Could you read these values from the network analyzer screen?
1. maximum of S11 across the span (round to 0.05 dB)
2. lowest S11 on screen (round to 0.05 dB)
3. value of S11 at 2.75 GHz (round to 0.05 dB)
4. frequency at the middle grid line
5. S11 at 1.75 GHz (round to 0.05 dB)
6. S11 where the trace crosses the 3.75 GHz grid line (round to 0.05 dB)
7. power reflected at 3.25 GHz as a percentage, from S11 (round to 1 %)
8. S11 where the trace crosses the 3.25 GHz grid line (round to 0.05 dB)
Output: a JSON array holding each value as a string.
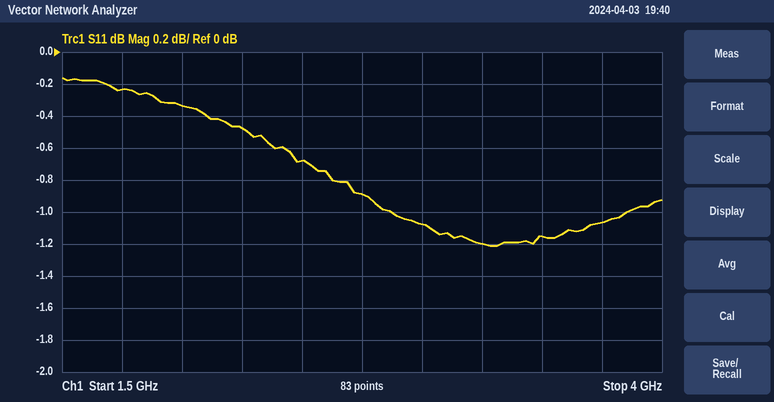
["-0.15 dB", "-1.20 dB", "-0.90 dB", "2.75 GHz", "-0.25 dB", "-1.05 dB", "76 %", "-1.20 dB"]
